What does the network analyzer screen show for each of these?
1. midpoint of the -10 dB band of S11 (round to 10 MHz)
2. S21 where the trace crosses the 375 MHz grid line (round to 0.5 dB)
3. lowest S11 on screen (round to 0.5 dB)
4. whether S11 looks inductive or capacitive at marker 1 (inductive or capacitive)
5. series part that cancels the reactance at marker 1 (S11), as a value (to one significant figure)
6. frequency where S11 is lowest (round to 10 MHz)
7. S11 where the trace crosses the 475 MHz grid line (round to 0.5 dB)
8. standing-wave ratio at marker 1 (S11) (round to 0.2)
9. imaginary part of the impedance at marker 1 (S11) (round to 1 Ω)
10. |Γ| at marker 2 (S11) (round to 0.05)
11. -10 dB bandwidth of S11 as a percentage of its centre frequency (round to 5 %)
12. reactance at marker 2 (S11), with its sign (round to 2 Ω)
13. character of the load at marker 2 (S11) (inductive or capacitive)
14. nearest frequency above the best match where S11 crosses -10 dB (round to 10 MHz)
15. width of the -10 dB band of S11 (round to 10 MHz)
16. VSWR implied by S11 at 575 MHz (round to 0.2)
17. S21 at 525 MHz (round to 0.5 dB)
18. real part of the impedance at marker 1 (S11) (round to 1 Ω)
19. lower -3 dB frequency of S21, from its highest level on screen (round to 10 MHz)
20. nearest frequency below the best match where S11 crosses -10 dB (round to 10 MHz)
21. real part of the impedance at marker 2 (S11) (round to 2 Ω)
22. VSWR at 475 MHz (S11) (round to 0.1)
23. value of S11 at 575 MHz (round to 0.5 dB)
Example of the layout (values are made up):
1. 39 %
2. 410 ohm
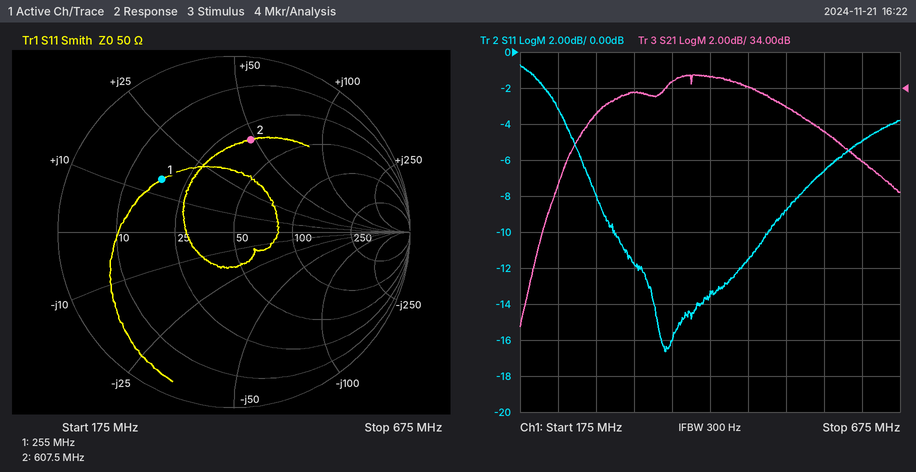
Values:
1. 400 MHz
2. 34.5 dB
3. -16.5 dB
4. inductive
5. 40 pF
6. 370 MHz
7. -11.5 dB
8. 3.0
9. +14 Ω
10. 0.55
11. 50 %
12. +48 Ω
13. inductive
14. 500 MHz
15. 200 MHz
16. 2.8
17. 33.0 dB
18. 18 Ω
19. 260 MHz
20. 300 MHz
21. 32 Ω
22. 1.7
23. -6.5 dB
